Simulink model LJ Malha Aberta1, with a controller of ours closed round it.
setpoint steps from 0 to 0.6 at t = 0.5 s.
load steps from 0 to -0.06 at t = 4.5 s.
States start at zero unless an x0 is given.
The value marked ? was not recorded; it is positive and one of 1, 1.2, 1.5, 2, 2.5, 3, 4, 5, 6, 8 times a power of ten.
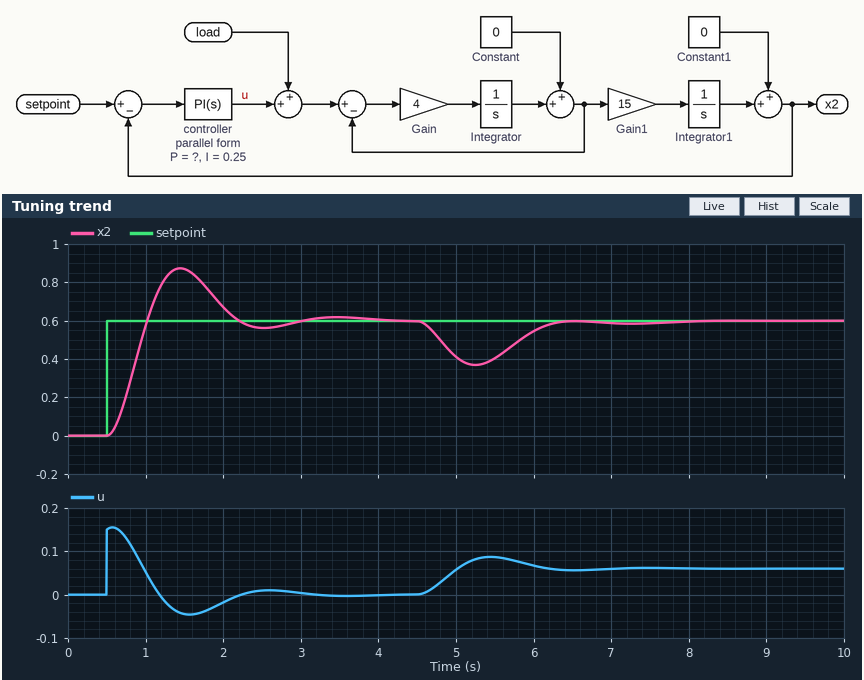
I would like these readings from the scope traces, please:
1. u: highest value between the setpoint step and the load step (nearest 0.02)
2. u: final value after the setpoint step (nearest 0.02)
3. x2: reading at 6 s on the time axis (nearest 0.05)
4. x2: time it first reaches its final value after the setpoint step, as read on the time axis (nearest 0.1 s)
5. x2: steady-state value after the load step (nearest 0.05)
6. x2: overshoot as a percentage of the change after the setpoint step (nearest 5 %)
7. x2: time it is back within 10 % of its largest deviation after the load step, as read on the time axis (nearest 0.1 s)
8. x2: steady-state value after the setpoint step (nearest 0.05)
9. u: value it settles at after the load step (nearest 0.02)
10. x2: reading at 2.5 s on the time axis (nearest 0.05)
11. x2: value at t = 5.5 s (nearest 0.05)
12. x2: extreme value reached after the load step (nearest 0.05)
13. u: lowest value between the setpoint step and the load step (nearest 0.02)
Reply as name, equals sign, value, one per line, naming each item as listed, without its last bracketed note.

u: highest value between the setpoint step and the load step = 0.16
u: final value after the setpoint step = 0.00
x2: reading at 6 s on the time axis = 0.55
x2: time it first reaches its final value after the setpoint step, as read on the time axis = 1.0 s
x2: steady-state value after the load step = 0.60
x2: overshoot as a percentage of the change after the setpoint step = 45 %
x2: time it is back within 10 % of its largest deviation after the load step, as read on the time axis = 6.2 s
x2: steady-state value after the setpoint step = 0.60
u: value it settles at after the load step = 0.06
x2: reading at 2.5 s on the time axis = 0.55
x2: value at t = 5.5 s = 0.40
x2: extreme value reached after the load step = 0.35
u: lowest value between the setpoint step and the load step = -0.04
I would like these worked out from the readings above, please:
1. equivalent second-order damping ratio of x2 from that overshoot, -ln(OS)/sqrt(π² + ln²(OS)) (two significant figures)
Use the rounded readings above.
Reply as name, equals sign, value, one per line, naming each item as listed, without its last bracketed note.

equivalent second-order damping ratio of x2 from that overshoot, -ln(OS)/sqrt(π² + ln²(OS)) = 0.25
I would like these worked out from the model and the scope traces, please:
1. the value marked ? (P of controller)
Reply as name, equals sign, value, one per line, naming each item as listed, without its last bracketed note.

the value marked ? = 0.25
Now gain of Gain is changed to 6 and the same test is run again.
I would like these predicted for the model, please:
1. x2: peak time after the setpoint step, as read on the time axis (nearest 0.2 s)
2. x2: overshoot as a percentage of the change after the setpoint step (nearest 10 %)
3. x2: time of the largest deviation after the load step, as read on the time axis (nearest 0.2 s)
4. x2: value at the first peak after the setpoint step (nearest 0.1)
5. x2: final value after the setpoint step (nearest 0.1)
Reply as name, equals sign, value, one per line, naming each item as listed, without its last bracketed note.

x2: peak time after the setpoint step, as read on the time axis = 1.4 s
x2: overshoot as a percentage of the change after the setpoint step = 30 %
x2: time of the largest deviation after the load step, as read on the time axis = 5.2 s
x2: value at the first peak after the setpoint step = 0.8
x2: final value after the setpoint step = 0.6
